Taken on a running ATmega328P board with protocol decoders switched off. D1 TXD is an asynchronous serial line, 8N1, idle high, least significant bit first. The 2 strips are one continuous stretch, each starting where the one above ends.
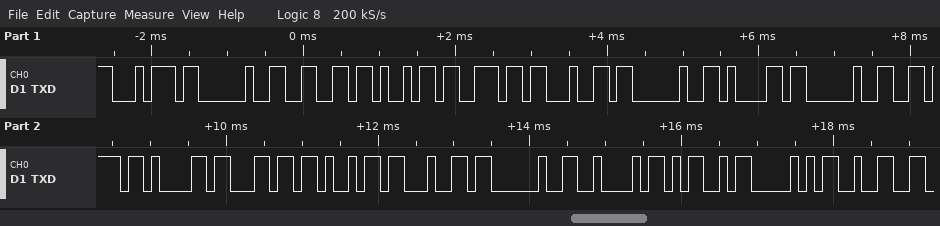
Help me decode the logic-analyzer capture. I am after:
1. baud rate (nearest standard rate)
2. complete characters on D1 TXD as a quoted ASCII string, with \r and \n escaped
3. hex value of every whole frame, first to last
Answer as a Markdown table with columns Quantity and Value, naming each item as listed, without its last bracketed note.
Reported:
| Quantity | Value |
|---|---|
| baud rate | 9600 baud |
| complete characters on D1 TXD as a quoted ASCII string, with \r and \n escaped | "t find a valid BMP2" |
| hex value of every whole frame, first to last | 0x74 0x20 0x66 0x69 0x6E 0x64 0x20 0x61 0x20 0x76 0x61 0x6C 0x69 0x64 0x20 0x42 0x4D 0x50 0x32 |
